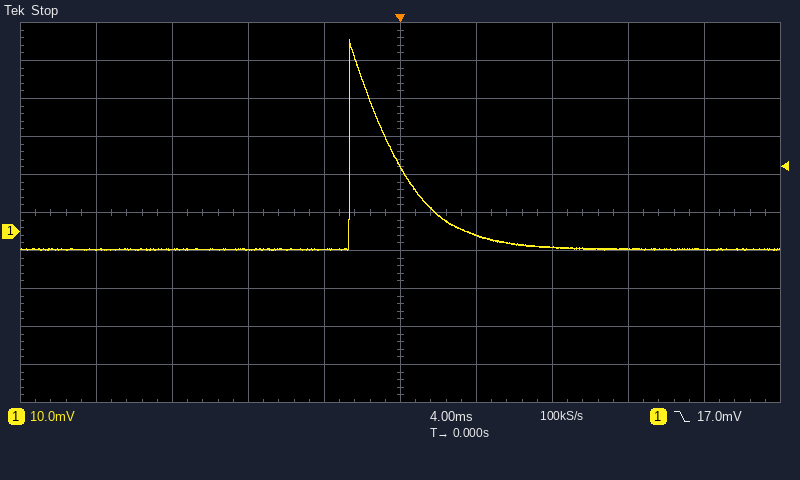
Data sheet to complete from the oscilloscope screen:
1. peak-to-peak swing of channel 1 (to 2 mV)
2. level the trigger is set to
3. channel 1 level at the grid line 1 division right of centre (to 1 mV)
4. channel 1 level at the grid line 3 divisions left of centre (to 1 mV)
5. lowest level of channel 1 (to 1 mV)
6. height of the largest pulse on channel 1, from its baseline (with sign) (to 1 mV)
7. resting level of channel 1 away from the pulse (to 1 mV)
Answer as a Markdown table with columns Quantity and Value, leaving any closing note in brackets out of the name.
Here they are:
| Quantity | Value |
|---|---|
| peak-to-peak swing of channel 1 | 56 mV |
| level the trigger is set to | 17.0 mV |
| channel 1 level at the grid line 1 division right of centre | -1 mV |
| channel 1 level at the grid line 3 divisions left of centre | -5 mV |
| lowest level of channel 1 | -5 mV |
| height of the largest pulse on channel 1, from its baseline (with sign) | +55 mV |
| resting level of channel 1 away from the pulse | -5 mV |
